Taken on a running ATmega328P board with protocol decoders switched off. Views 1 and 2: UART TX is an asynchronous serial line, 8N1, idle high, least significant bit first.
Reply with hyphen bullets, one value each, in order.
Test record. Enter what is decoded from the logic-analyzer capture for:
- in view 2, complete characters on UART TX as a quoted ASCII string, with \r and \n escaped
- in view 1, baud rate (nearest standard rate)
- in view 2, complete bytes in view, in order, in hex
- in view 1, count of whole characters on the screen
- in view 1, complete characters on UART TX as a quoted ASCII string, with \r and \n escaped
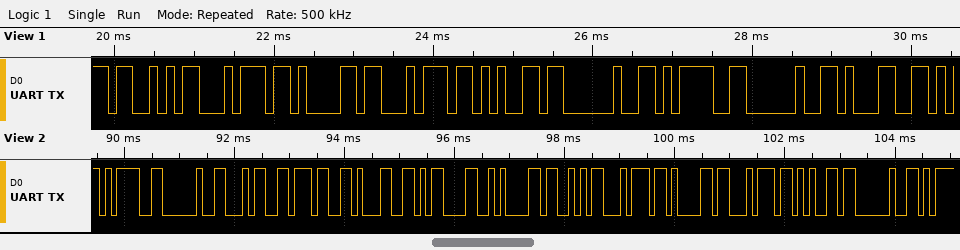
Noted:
- "= 471\r\nState "
- 9600 baud
- 3D 20 34 37 31 0D 0A 53 74 61 74 65 20
- 9
- "State = 1"
